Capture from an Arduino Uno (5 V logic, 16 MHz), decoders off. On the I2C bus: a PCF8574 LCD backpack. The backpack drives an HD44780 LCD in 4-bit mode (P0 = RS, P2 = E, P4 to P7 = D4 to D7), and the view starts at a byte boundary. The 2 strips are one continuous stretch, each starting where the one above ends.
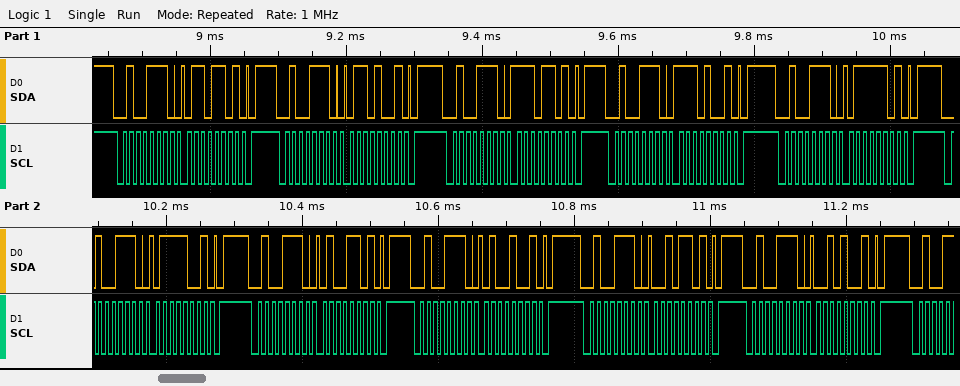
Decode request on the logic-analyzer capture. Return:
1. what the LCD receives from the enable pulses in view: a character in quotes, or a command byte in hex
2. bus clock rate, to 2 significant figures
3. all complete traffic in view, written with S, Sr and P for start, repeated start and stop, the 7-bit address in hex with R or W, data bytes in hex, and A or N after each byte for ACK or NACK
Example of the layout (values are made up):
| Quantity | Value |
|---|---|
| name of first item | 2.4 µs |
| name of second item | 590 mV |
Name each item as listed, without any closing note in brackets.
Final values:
| Quantity | Value |
|---|---|
| what the LCD receives from the enable pulses in view: a character in quotes, or a command byte in hex | 'n' 't' |
| bus clock rate, to 2 significant figures | 100 kHz |
| all complete traffic in view, written with S, Sr and P for start, repeated start and stop, the 7-bit address in hex with R or W, data bytes in hex, and A or N after each byte for ACK or NACK | S 27W A 6D A P S 27W A 69 A P S 27W A ED A P S 27W A E9 A P S 27W A 7D A P S 27W A 79 A P S 27W A 4D A P S 27W A 49 A P S 27W A 2D A P S 27W A 29 A P |
